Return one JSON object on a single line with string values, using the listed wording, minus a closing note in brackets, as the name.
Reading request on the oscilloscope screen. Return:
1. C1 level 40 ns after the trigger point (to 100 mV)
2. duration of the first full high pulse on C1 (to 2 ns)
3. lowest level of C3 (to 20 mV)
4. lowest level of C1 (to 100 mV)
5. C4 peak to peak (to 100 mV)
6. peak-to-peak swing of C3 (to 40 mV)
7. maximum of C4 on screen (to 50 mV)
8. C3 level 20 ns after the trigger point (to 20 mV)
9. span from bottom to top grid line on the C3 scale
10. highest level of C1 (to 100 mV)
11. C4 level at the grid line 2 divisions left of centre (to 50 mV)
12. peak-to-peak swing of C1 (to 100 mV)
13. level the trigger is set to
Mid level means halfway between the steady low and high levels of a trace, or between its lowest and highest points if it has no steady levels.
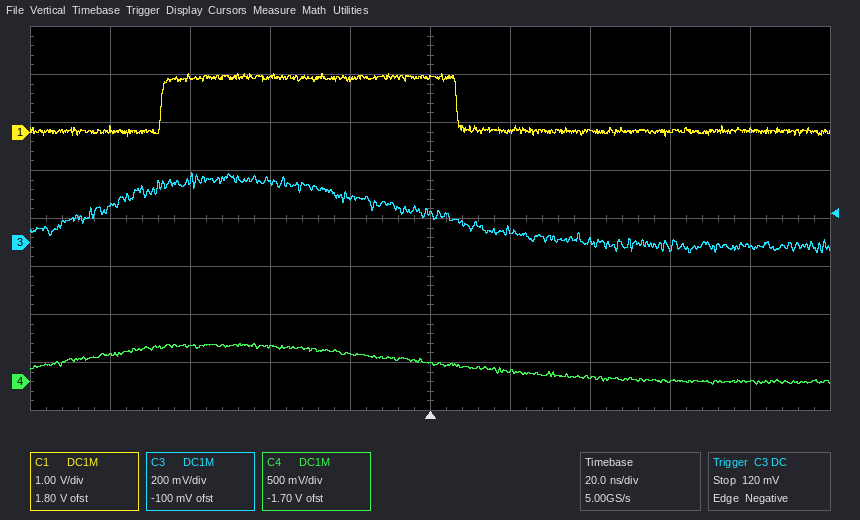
{"C1 level 40 ns after the trigger point": "0.0 V", "duration of the first full high pulse on C1": "74 ns", "lowest level of C3": "-40 mV", "lowest level of C1": "-100 mV", "C4 peak to peak": "400 mV", "peak-to-peak swing of C3": "320 mV", "maximum of C4 on screen": "400 mV", "C3 level 20 ns after the trigger point": "60 mV", "span from bottom to top grid line on the C3 scale": "1.6 V", "highest level of C1": "1.2 V", "C4 level at the grid line 2 divisions left of centre": "350 mV", "peak-to-peak swing of C1": "1.3 V", "level the trigger is set to": "120 mV"}
